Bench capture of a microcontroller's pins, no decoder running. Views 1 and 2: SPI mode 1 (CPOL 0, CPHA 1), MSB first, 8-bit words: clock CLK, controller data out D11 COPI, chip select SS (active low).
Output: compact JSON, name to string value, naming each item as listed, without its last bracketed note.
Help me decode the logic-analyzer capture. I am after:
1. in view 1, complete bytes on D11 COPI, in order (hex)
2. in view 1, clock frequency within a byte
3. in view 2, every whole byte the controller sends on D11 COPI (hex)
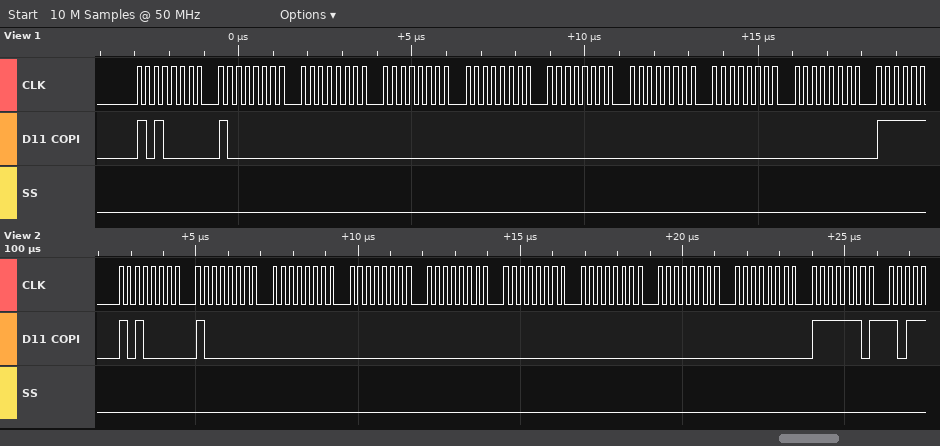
{"in view 1, complete bytes on D11 COPI, in order": "A0 80 00 00 00 00 00 00 00", "in view 1, clock frequency within a byte": "4 MHz", "in view 2, every whole byte the controller sends on D11 COPI": "A0 80 00 00 00 00 00 00 00 FD"}
